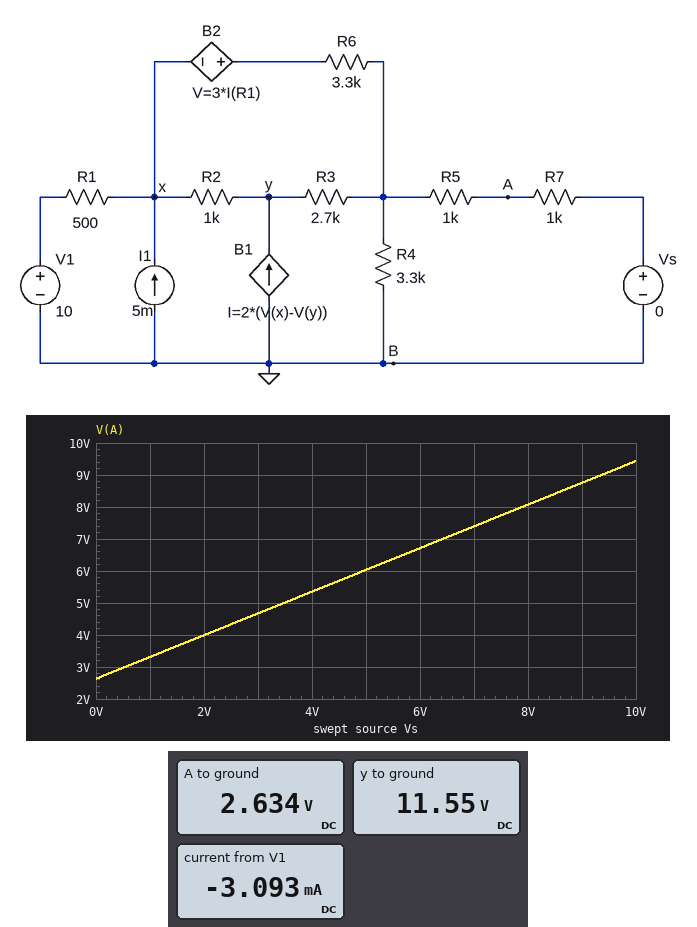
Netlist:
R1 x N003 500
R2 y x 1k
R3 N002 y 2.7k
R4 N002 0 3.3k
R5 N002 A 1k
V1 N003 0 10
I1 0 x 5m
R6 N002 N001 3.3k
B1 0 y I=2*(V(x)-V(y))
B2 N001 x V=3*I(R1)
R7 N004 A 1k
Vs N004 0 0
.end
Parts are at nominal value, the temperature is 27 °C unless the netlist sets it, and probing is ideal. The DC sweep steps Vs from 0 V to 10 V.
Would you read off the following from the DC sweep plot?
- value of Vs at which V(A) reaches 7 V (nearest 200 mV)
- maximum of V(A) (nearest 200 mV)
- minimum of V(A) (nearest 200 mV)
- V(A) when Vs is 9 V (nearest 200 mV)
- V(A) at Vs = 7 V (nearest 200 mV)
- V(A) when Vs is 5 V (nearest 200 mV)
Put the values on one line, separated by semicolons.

6.4 V; 9.4 V; 2.6 V; 8.8 V; 7.4 V; 6.0 V
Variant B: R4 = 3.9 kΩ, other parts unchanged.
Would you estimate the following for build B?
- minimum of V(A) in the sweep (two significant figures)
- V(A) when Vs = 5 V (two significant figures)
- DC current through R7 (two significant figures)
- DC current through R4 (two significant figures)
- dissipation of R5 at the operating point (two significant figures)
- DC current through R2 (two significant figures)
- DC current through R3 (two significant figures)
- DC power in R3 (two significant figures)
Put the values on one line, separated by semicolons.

2.7 V; 6.2 V; 2.7 mA; 1.4 mA; 7.4 mW; 1.1 µA; 2.3 mA; 14 mW
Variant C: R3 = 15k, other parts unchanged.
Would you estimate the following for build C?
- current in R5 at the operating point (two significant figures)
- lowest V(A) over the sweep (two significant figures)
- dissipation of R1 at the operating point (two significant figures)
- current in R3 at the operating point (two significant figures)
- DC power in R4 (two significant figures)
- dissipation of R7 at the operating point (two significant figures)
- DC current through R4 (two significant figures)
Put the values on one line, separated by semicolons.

1.8 mA; 1.8 V; 3.5 mW; 520 µA; 3.9 mW; 3.2 mW; 1.1 mA
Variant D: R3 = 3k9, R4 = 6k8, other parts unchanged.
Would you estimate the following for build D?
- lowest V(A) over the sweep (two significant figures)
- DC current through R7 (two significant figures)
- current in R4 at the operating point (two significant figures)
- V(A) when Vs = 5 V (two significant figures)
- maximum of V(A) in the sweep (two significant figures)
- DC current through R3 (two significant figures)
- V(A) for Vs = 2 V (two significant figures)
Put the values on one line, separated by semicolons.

2.7 V; 2.7 mA; 790 µA; 6.3 V; 9.9 V; 1.6 mA; 4.1 V
